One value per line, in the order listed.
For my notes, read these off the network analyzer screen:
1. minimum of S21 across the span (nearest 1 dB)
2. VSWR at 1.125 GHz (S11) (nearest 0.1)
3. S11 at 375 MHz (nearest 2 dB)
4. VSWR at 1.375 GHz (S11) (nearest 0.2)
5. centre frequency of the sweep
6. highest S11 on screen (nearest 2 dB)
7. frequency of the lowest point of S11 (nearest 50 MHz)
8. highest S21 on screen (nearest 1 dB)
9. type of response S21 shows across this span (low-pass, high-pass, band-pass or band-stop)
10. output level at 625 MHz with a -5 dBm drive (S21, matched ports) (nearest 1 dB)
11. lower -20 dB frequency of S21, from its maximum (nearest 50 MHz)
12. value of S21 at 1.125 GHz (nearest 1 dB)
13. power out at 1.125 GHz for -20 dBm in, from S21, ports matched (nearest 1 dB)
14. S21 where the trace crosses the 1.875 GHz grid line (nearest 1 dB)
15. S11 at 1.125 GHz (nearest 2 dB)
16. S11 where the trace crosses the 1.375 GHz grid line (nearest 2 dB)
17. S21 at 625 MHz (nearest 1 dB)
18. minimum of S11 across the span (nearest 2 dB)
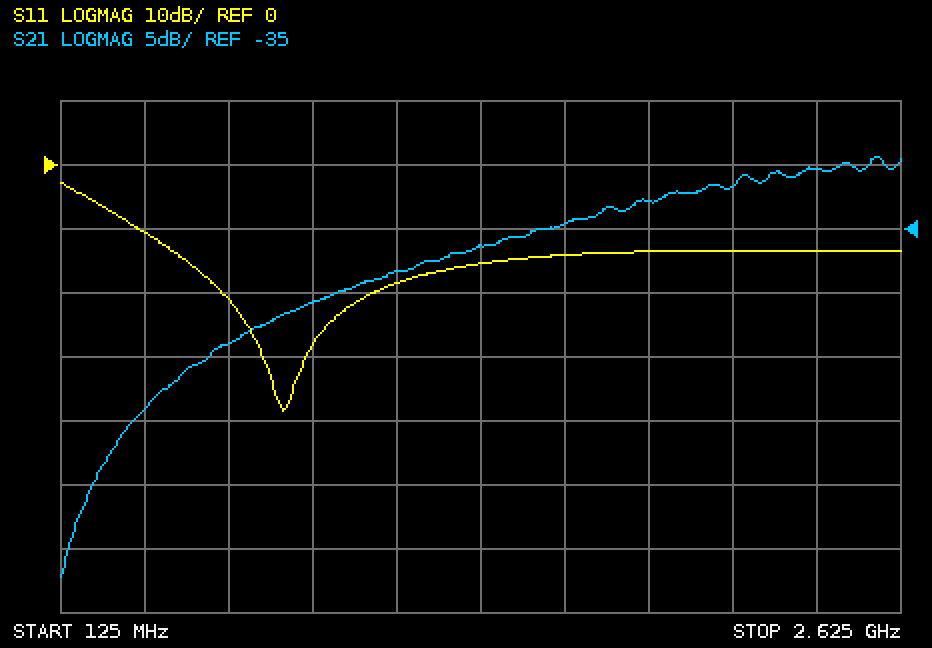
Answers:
-62 dB
1.3
-10 dB
1.4
1.375 GHz
-2 dB
800 MHz
-29 dB
high-pass
-49 dBm
350 MHz
-38 dB
-58 dBm
-33 dB
-18 dB
-16 dB
-44 dB
-38 dB
